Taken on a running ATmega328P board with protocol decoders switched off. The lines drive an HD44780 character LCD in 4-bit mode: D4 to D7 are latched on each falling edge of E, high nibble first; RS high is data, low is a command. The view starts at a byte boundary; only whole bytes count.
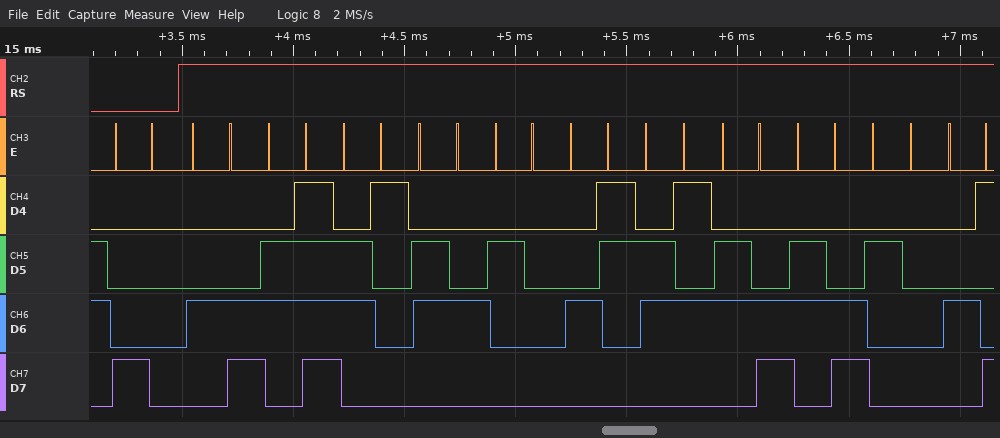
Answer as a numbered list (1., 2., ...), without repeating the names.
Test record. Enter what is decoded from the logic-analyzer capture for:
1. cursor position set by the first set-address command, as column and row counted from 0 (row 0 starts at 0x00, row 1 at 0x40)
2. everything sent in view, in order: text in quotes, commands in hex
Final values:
1. column 0, row 0
2. 0x80 "Load Cell I"
